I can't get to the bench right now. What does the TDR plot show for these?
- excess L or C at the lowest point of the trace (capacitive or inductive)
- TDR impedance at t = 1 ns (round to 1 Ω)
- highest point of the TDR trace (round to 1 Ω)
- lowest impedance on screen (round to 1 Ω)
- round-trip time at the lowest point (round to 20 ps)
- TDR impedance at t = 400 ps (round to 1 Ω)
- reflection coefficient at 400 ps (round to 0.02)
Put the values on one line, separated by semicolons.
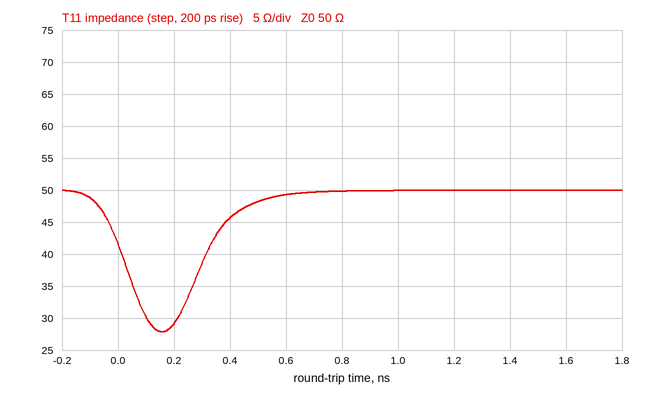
capacitive; 50 Ω; 50 Ω; 28 Ω; 160 ps; 46 Ω; -0.04
